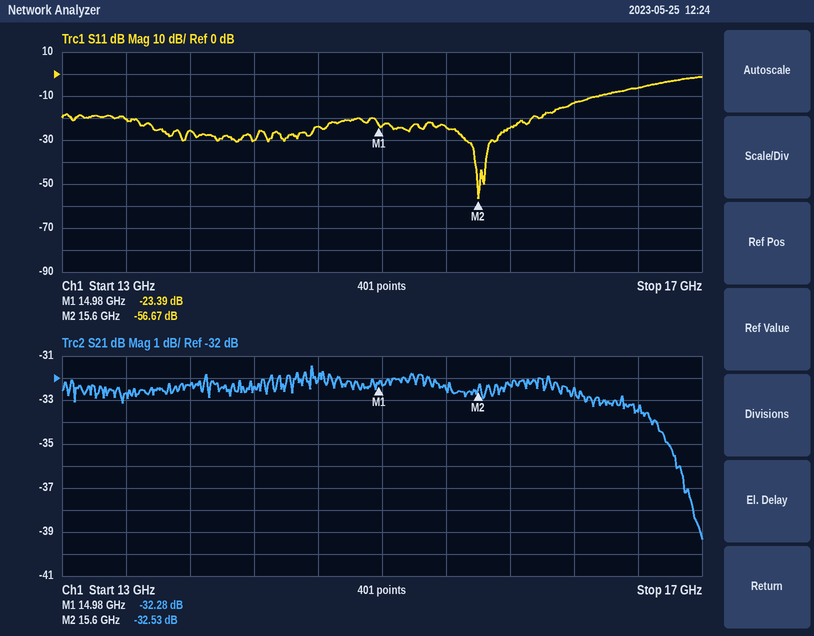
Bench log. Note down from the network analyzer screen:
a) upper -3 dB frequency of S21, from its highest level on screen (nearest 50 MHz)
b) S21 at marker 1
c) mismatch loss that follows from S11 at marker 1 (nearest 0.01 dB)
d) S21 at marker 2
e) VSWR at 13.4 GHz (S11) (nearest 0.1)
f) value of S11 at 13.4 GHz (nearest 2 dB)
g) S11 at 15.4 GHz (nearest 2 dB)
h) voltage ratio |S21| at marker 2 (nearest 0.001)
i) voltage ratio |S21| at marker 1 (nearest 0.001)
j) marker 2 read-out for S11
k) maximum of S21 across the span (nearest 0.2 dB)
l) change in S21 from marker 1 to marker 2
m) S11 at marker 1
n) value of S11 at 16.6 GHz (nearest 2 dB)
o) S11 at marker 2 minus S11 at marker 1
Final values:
16.75 GHz
-32.28 dB
0.02 dB
-32.53 dB
1.2
-20 dB
-24 dB
0.024
0.024
-56.67 dB
-31.4 dB
-0.25 dB
-23.39 dB
-6 dB
-33.28 dB
